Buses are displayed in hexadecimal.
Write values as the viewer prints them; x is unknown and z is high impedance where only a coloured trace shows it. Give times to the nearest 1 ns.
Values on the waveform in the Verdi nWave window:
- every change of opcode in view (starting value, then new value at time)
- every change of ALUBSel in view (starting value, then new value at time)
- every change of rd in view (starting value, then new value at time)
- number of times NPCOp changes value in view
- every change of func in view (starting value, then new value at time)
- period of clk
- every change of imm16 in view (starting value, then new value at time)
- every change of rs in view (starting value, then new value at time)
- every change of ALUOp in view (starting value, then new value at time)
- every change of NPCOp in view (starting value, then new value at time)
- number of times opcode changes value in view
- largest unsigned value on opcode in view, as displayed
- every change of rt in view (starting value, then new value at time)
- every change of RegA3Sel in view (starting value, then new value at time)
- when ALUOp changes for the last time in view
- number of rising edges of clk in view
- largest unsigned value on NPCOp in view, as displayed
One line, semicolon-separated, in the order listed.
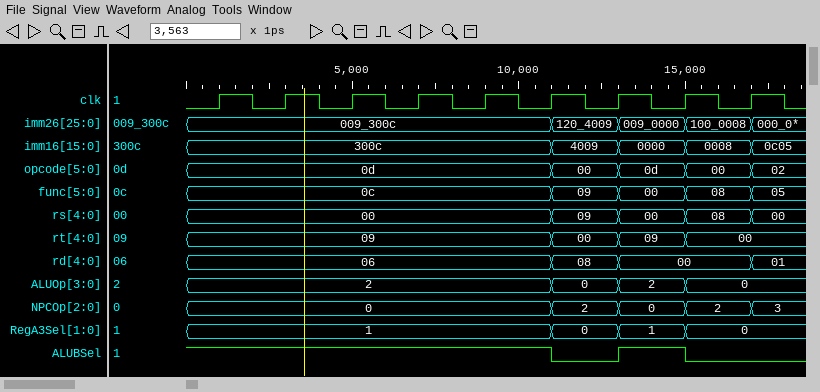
0d, 00 at 11 ns, 0d at 13 ns, 00 at 15 ns, 02 at 17 ns; 1, 0 at 11 ns, 1 at 13 ns, 0 at 15 ns; 06, 08 at 11 ns, 00 at 13 ns, 01 at 17 ns; 4; 0c, 09 at 11 ns, 00 at 13 ns, 08 at 15 ns, 05 at 17 ns; 2 ns; 300c, 4009 at 11 ns, 0000 at 13 ns, 0008 at 15 ns, 0c05 at 17 ns; 00, 09 at 11 ns, 00 at 13 ns, 08 at 15 ns, 00 at 17 ns; 2, 0 at 11 ns, 2 at 13 ns, 0 at 15 ns; 0, 2 at 11 ns, 0 at 13 ns, 2 at 15 ns, 3 at 17 ns; 4; 0d; 09, 00 at 11 ns, 09 at 13 ns, 00 at 15 ns; 1, 0 at 11 ns, 1 at 13 ns, 0 at 15 ns; 15 ns; 9; 3
